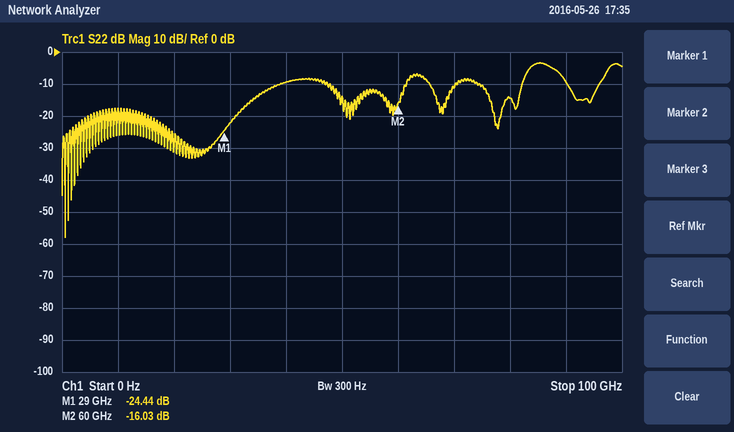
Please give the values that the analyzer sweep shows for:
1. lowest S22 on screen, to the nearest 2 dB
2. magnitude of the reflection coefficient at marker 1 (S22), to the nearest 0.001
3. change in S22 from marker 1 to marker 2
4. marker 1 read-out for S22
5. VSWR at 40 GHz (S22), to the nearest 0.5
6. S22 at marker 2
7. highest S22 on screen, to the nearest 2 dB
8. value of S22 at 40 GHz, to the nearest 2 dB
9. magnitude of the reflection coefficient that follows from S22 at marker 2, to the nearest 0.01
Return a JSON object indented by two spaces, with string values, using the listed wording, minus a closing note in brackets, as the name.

{
  "lowest S22 on screen, to the nearest 2 dB": "-58 dB",
  "magnitude of the reflection coefficient at marker 1 (S22), to the nearest 0.001": "0.060",
  "change in S22 from marker 1 to marker 2": "8.41 dB",
  "marker 1 read-out for S22": "-24.44 dB",
  "VSWR at 40 GHz (S22), to the nearest 0.5": "2.0",
  "S22 at marker 2": "-16.03 dB",
  "highest S22 on screen, to the nearest 2 dB": "-4 dB",
  "value of S22 at 40 GHz, to the nearest 2 dB": "-10 dB",
  "magnitude of the reflection coefficient that follows from S22 at marker 2, to the nearest 0.01": "0.16"
}
